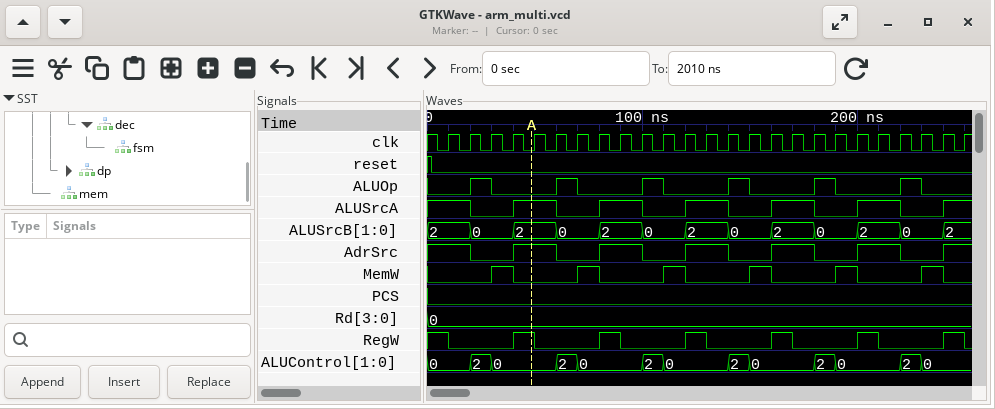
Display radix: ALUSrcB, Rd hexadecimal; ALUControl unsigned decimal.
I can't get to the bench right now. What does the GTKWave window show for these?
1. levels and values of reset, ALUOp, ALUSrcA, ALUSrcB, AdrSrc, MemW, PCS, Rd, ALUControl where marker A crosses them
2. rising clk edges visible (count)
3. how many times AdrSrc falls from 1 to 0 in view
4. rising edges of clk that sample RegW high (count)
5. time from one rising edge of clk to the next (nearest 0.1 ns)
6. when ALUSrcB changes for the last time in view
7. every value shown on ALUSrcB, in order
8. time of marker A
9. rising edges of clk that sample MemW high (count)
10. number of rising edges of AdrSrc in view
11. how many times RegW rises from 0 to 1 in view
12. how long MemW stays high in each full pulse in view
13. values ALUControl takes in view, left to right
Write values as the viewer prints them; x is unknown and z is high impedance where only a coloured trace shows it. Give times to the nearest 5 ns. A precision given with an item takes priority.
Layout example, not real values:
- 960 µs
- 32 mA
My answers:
- reset=0, ALUOp=0, ALUSrcA=1, ALUSrcB=2, AdrSrc=1, MemW=0, PCS=0, Rd=0, ALUControl=0
- 25
- 6
- 7
- 10 ns
- 240 ns
- 2, 0, 2, 0, 2, 0, 2, 0, 2, 0, 2, 0, 2
- 50 ns
- 6
- 6
- 6
- 10 ns, 10 ns, 10 ns, 10 ns, 10 ns, 10 ns
- 0, 2, 0, 2, 0, 2, 0, 2, 0, 2, 0, 2, 0
